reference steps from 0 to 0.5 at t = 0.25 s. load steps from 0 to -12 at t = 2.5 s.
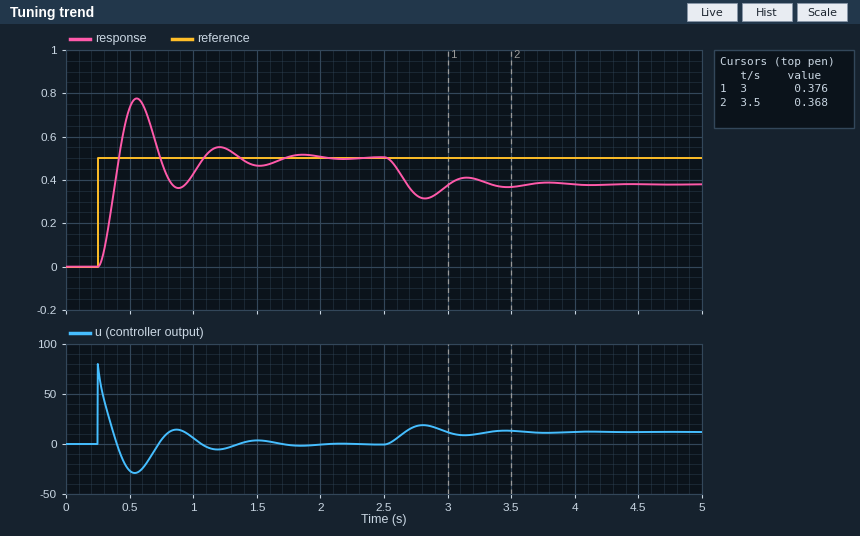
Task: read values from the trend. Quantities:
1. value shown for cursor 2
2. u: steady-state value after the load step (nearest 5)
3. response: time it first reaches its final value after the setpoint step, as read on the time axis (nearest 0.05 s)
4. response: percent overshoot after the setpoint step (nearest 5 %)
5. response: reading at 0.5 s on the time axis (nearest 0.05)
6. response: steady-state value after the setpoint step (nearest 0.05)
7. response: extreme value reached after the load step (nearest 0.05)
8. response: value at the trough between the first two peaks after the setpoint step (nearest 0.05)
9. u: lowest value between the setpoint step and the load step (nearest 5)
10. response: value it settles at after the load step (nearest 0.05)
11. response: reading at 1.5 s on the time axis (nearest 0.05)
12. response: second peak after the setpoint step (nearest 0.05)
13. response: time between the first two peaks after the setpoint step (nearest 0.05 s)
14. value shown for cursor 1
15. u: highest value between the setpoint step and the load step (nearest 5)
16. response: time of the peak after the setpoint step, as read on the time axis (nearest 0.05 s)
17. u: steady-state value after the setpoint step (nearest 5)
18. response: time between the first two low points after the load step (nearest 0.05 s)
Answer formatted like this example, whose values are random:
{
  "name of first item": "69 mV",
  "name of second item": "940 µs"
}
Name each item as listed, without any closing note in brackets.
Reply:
{
  "value shown for cursor 2": "0.368",
  "u: steady-state value after the load step": "10",
  "response: time it first reaches its final value after the setpoint step, as read on the time axis": "0.40 s",
  "response: percent overshoot after the setpoint step": "55 %",
  "response: reading at 0.5 s on the time axis": "0.75",
  "response: steady-state value after the setpoint step": "0.50",
  "response: extreme value reached after the load step": "0.30",
  "response: value at the trough between the first two peaks after the setpoint step": "0.35",
  "u: lowest value between the setpoint step and the load step": "-30",
  "response: value it settles at after the load step": "0.40",
  "response: reading at 1.5 s on the time axis": "0.45",
  "response: second peak after the setpoint step": "0.55",
  "response: time between the first two peaks after the setpoint step": "0.65 s",
  "value shown for cursor 1": "0.376",
  "u: highest value between the setpoint step and the load step": "80",
  "response: time of the peak after the setpoint step, as read on the time axis": "0.55 s",
  "u: steady-state value after the setpoint step": "0",
  "response: time between the first two low points after the load step": "0.65 s"
}
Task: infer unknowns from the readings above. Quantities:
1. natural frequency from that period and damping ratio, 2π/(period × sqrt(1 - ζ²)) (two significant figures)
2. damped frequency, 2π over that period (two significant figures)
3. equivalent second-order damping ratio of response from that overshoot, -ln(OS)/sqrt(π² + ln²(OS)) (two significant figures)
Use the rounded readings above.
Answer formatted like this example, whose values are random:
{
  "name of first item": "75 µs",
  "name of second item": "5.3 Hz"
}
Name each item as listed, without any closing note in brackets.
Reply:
{
  "natural frequency from that period and damping ratio, 2π/(period × sqrt(1 - ζ²))": "9.8 rad/s",
  "damped frequency, 2π over that period": "9.7 rad/s",
  "equivalent second-order damping ratio of response from that overshoot, -ln(OS)/sqrt(π² + ln²(OS))": "0.19"
}
